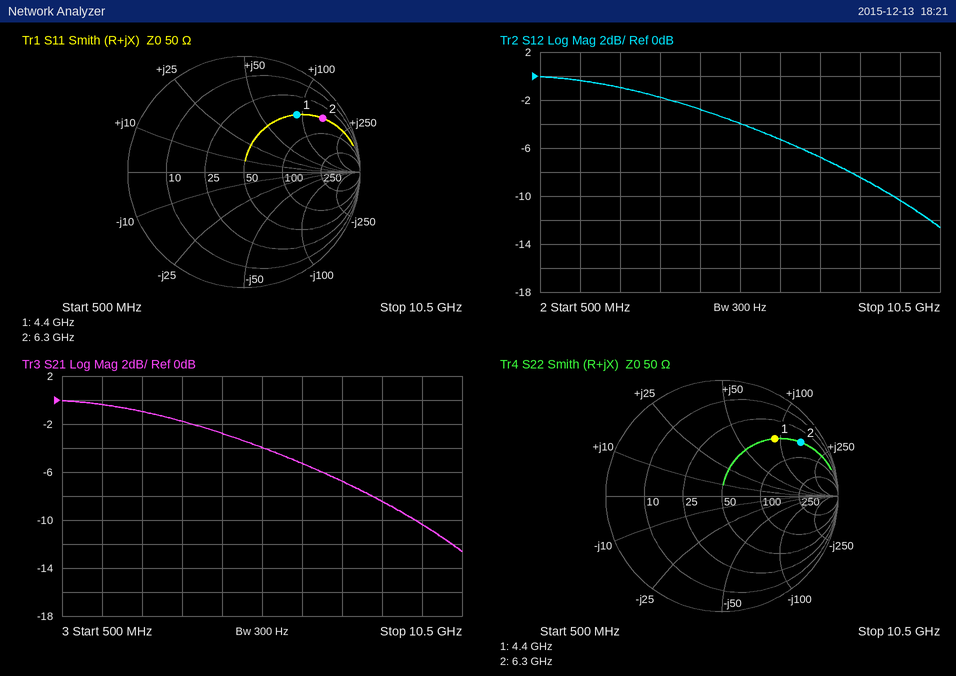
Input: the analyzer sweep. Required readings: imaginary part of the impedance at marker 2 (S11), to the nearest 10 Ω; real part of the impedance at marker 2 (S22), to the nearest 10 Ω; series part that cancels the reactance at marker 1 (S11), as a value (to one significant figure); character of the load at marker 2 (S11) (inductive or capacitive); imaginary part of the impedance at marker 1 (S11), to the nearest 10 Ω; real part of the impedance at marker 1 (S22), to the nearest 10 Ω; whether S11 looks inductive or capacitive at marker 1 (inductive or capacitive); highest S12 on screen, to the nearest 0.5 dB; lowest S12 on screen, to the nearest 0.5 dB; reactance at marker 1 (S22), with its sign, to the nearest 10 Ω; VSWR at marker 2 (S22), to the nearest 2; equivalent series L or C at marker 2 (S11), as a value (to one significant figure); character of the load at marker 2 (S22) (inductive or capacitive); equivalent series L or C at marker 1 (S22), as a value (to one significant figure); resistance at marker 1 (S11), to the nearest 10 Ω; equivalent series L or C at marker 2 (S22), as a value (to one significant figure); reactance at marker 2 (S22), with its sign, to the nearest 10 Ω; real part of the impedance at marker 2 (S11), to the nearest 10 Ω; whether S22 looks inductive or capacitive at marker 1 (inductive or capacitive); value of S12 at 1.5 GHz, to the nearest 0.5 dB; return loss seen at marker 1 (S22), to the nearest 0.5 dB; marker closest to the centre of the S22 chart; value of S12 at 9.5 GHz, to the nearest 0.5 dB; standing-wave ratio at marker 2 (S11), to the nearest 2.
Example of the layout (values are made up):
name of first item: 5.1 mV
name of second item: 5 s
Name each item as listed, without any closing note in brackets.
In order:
imaginary part of the impedance at marker 2 (S11), to the nearest 10 Ω: +150 Ω
real part of the impedance at marker 2 (S22), to the nearest 10 Ω: 50 Ω
series part that cancels the reactance at marker 1 (S11), as a value: 400 fF
character of the load at marker 2 (S11): inductive
imaginary part of the impedance at marker 1 (S11), to the nearest 10 Ω: +90 Ω
real part of the impedance at marker 1 (S22), to the nearest 10 Ω: 50 Ω
whether S11 looks inductive or capacitive at marker 1: inductive
highest S12 on screen, to the nearest 0.5 dB: 0.0 dB
lowest S12 on screen, to the nearest 0.5 dB: -12.5 dB
reactance at marker 1 (S22), with its sign, to the nearest 10 Ω: +90 Ω
VSWR at marker 2 (S22), to the nearest 2: 10
equivalent series L or C at marker 2 (S11), as a value: 4 nH
character of the load at marker 2 (S22): inductive
equivalent series L or C at marker 1 (S22), as a value: 3 nH
resistance at marker 1 (S11), to the nearest 10 Ω: 50 Ω
equivalent series L or C at marker 2 (S22), as a value: 4 nH
reactance at marker 2 (S22), with its sign, to the nearest 10 Ω: +150 Ω
real part of the impedance at marker 2 (S11), to the nearest 10 Ω: 50 Ω
whether S22 looks inductive or capacitive at marker 1: inductive
value of S12 at 1.5 GHz, to the nearest 0.5 dB: -0.5 dB
return loss seen at marker 1 (S22), to the nearest 0.5 dB: 3.5 dB
marker closest to the centre of the S22 chart: marker 1
value of S12 at 9.5 GHz, to the nearest 0.5 dB: -10.5 dB
standing-wave ratio at marker 2 (S11), to the nearest 2: 10
